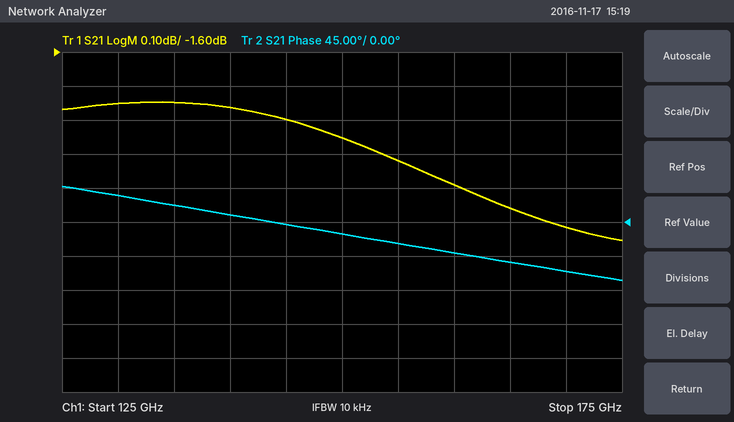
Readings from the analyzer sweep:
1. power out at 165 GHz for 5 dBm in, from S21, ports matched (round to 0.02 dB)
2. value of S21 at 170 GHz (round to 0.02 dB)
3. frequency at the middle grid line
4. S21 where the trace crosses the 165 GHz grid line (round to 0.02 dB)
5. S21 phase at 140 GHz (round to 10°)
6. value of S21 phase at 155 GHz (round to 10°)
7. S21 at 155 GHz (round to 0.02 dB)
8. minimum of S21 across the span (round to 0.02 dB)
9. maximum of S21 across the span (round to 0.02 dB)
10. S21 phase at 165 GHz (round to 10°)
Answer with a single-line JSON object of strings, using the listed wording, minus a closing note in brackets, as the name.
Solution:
{"power out at 165 GHz for 5 dBm in, from S21, ports matched": "2.94 dBm", "value of S21 at 170 GHz": "-2.12 dB", "frequency at the middle grid line": "150 GHz", "S21 where the trace crosses the 165 GHz grid line": "-2.06 dB", "S21 phase at 140 GHz": "10°", "value of S21 phase at 155 GHz": "-30°", "S21 at 155 GHz": "-1.92 dB", "minimum of S21 across the span": "-2.16 dB", "maximum of S21 across the span": "-1.74 dB", "S21 phase at 165 GHz": "-50°"}
